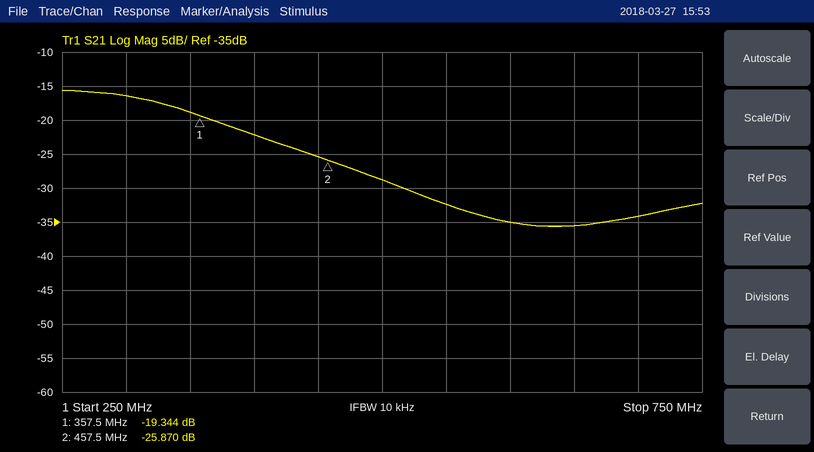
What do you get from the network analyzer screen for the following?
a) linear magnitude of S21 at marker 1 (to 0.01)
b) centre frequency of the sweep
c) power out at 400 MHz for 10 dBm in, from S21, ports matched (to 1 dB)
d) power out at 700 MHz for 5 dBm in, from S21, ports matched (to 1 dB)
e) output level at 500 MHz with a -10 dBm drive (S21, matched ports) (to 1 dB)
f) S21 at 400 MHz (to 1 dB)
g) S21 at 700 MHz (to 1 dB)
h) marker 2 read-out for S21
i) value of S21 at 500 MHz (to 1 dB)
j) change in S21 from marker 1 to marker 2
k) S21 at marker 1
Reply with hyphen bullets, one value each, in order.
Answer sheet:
- 0.11
- 500 MHz
- -12 dBm
- -29 dBm
- -39 dBm
- -22 dB
- -34 dB
- -25.870 dB
- -29 dB
- -6.526 dB
- -19.344 dB
